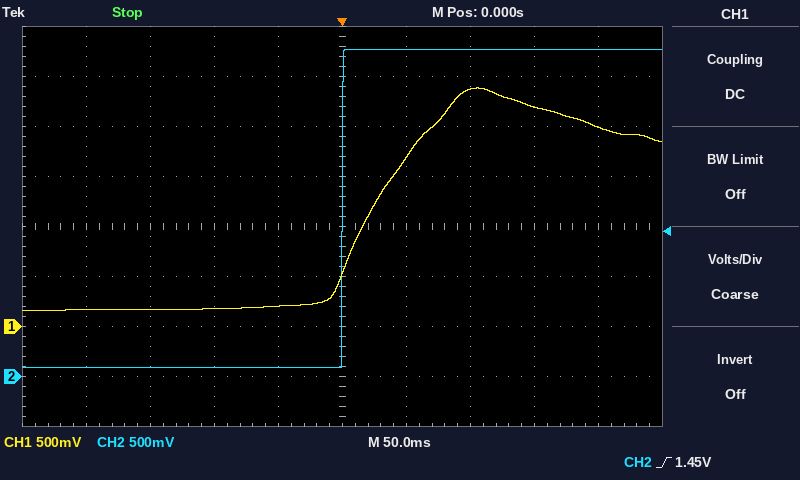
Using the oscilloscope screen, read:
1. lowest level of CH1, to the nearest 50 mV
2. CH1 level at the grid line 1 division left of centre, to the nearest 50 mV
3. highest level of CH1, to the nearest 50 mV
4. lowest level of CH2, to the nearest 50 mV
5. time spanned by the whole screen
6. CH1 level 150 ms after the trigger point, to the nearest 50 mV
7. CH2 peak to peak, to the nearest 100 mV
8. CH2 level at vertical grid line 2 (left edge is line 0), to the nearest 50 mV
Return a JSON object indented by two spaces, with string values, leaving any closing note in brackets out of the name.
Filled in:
{
  "lowest level of CH1, to the nearest 50 mV": "150 mV",
  "CH1 level at the grid line 1 division left of centre, to the nearest 50 mV": "200 mV",
  "highest level of CH1, to the nearest 50 mV": "2.40 V",
  "lowest level of CH2, to the nearest 50 mV": "100 mV",
  "time spanned by the whole screen": "500 ms",
  "CH1 level 150 ms after the trigger point, to the nearest 50 mV": "2.20 V",
  "CH2 peak to peak, to the nearest 100 mV": "3.20 V",
  "CH2 level at vertical grid line 2 (left edge is line 0), to the nearest 50 mV": "100 mV"
}
